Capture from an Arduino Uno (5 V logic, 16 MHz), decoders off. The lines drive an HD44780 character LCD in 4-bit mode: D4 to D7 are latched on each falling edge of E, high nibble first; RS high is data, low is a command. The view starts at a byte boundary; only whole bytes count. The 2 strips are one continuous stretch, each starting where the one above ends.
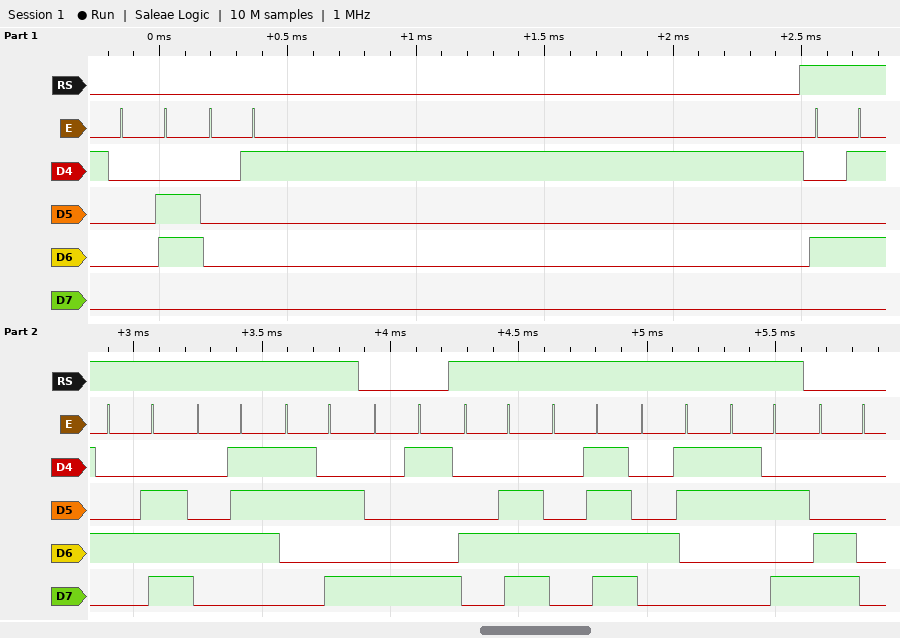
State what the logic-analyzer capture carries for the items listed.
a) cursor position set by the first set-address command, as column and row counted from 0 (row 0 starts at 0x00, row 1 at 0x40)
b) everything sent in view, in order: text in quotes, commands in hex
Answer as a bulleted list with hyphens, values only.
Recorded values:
- column 9, row 0
- 0x06 0x01 "ENG:" 0x89 "NOC:" 0xC0
